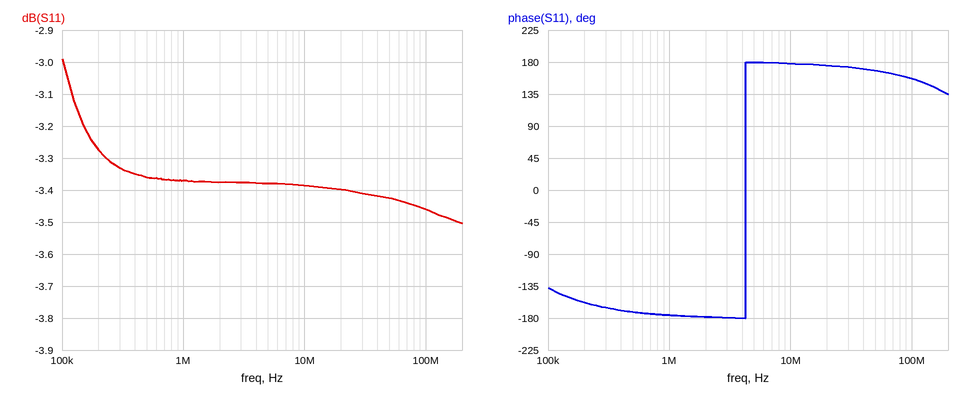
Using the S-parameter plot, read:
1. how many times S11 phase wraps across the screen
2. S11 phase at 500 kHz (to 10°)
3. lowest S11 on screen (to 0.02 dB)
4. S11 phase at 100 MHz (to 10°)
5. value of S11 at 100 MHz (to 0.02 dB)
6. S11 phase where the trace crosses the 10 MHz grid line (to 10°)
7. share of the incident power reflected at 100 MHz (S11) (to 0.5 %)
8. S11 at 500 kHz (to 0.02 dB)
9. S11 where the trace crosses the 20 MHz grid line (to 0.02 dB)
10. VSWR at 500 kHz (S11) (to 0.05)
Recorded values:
1
-170°
-3.50 dB
160°
-3.46 dB
180°
45.0 %
-3.36 dB
-3.40 dB
5.25
